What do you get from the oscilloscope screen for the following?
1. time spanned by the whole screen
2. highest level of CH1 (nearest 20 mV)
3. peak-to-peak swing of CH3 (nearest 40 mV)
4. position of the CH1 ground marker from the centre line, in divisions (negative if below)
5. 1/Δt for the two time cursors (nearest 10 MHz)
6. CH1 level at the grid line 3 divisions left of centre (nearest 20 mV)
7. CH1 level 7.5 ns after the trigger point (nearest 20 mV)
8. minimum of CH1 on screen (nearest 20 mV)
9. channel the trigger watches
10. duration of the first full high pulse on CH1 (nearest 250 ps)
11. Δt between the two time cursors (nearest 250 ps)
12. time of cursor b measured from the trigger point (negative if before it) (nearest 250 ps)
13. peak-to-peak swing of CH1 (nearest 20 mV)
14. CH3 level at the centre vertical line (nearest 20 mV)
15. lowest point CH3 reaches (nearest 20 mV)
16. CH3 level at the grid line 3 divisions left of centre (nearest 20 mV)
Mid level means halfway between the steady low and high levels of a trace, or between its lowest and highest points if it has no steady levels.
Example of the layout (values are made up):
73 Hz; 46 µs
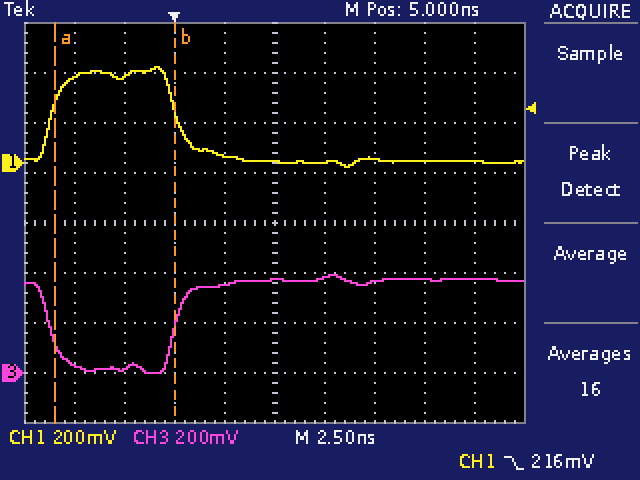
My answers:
25 ns; 380 mV; 400 mV; +1.2 div; 170 MHz; 340 mV; 0 mV; -20 mV; CH1; 6.25 ns; 6.00 ns; 0.00 ns; 400 mV; 380 mV; 0 mV; 20 mV
